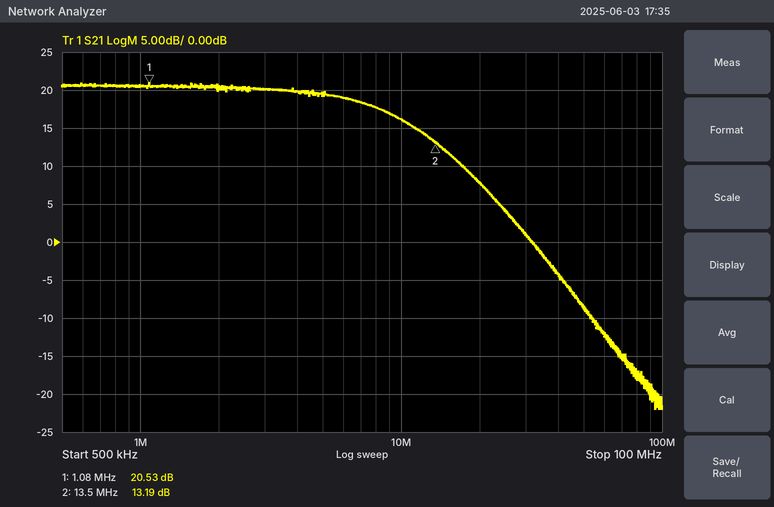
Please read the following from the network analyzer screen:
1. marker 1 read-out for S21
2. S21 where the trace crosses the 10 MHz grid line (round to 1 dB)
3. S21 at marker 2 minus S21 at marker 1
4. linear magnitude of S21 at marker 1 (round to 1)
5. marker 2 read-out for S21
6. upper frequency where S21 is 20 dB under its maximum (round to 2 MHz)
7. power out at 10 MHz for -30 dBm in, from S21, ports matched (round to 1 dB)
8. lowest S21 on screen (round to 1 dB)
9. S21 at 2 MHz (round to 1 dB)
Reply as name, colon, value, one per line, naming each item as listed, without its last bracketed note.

marker 1 read-out for S21: 20.53 dB
S21 where the trace crosses the 10 MHz grid line: 16 dB
S21 at marker 2 minus S21 at marker 1: -7.34 dB
linear magnitude of S21 at marker 1: 11
marker 2 read-out for S21: 13.19 dB
upper frequency where S21 is 20 dB under its maximum: 30 MHz
power out at 10 MHz for -30 dBm in, from S21, ports matched: -14 dBm
lowest S21 on screen: -22 dB
S21 at 2 MHz: 20 dB
